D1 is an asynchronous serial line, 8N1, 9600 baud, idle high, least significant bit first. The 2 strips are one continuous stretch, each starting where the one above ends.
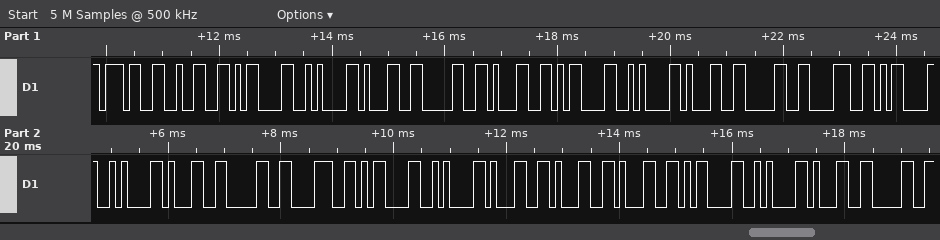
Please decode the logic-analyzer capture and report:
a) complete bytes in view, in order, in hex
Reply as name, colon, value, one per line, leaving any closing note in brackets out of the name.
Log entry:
complete bytes in view, in order, in hex: 0x37 0x32 0x0D 0x0A 0x31 0x30 0x31 0x0D 0x0A 0x31 0x30 0x38 0x0D 0x0A 0x31 0x30 0x38 0x0D 0x0A 0x31 0x31 0x31 0x0D 0x0A 0x31 0x30
